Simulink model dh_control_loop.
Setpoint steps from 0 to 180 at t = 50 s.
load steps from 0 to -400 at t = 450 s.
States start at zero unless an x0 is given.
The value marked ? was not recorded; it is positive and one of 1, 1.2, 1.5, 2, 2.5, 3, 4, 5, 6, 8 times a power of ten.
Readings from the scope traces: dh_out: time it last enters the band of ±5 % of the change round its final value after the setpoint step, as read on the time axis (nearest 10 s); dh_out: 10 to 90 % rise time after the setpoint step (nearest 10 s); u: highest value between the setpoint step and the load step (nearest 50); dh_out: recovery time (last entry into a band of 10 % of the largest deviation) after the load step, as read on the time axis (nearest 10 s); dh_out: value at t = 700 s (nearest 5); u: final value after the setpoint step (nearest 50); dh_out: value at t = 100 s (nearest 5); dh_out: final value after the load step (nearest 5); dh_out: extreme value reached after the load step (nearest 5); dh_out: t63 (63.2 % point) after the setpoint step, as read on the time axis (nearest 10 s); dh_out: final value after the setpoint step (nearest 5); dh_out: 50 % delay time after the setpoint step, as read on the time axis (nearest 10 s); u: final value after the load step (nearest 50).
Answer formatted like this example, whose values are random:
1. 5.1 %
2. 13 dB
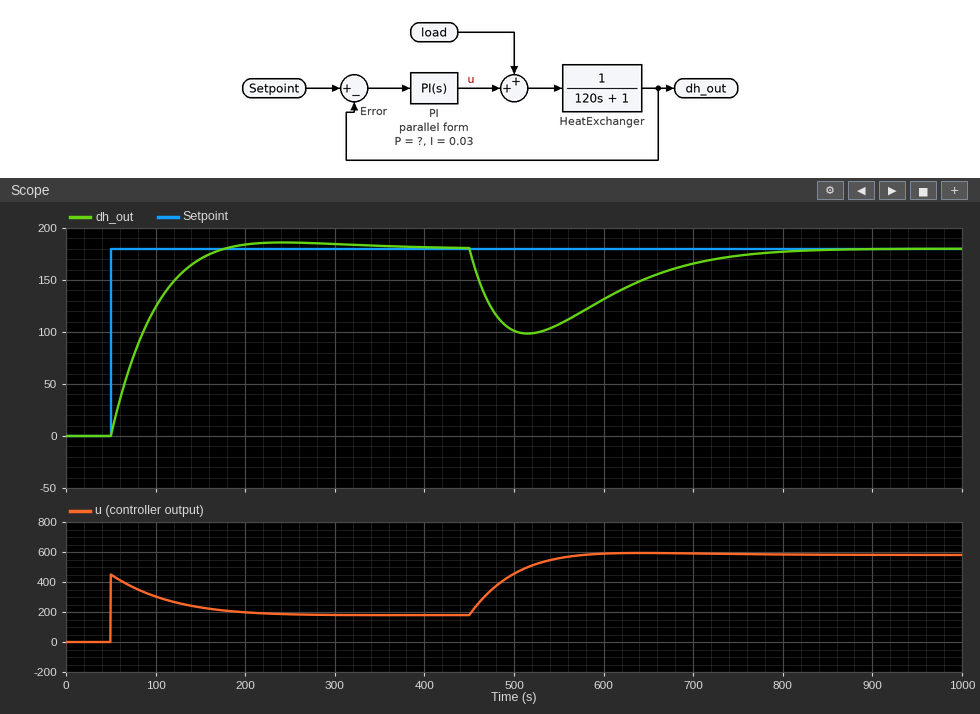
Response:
1. 150 s
2. 80 s
3. 450
4. 740 s
5. 165
6. 200
7. 125
8. 180
9. 100
10. 90 s
11. 180
12. 80 s
13. 600
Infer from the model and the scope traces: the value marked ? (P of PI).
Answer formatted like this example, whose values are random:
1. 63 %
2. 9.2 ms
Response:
1. 2.5
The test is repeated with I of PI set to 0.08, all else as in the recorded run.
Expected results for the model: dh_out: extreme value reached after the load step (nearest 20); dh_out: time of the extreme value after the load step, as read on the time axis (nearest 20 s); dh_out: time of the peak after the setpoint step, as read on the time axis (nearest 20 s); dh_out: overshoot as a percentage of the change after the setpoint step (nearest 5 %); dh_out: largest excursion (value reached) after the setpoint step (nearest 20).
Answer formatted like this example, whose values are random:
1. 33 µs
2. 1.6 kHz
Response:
1. 120
2. 500 s
3. 160 s
4. 20 %
5. 220
